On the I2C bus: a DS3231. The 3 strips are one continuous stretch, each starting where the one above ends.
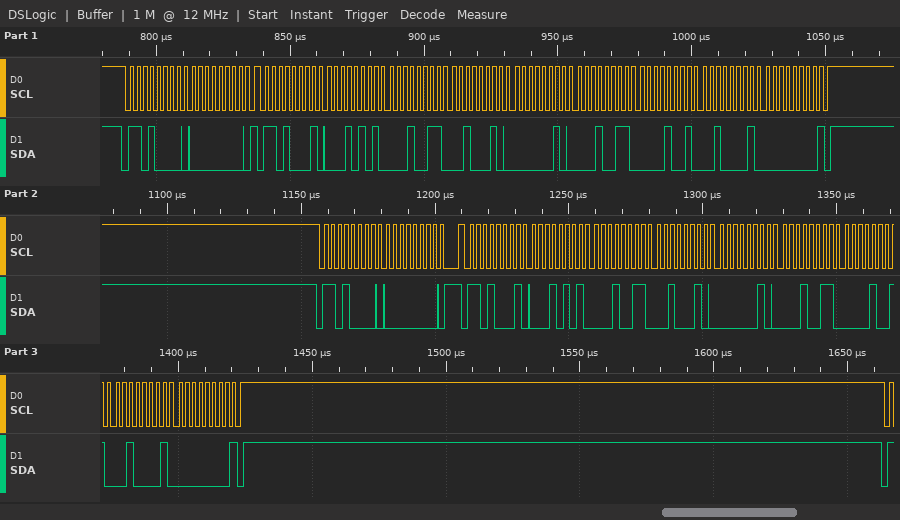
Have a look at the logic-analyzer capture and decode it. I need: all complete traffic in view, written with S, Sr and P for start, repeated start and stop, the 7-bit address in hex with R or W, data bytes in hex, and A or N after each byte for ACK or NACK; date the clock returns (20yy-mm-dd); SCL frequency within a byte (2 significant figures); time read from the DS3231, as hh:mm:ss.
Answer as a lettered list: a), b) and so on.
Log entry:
a) S 68W A 00 A Sr 68R A 15 A 13 A 22 A 02 A 13 A 09 A 21 A 00 N P S 68W A 00 A Sr 68R A 15 A 13 A 22 A 02 A 13 A 09 A 21 A 00 N P
b) 2021-09-13
c) 400 kHz
d) 22:13:15
